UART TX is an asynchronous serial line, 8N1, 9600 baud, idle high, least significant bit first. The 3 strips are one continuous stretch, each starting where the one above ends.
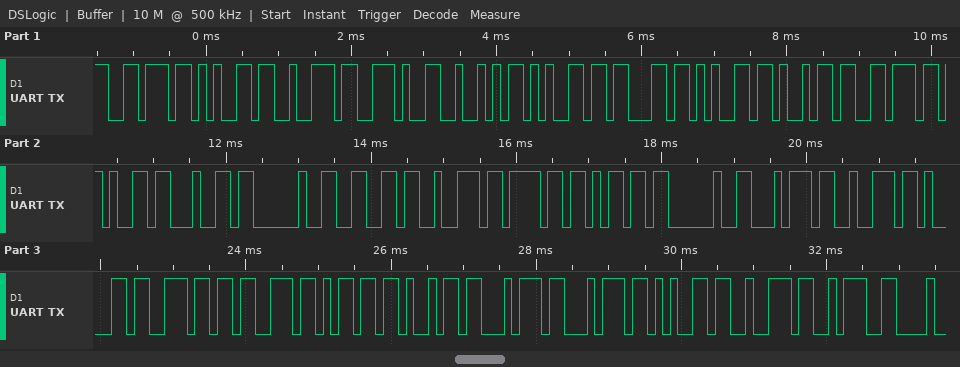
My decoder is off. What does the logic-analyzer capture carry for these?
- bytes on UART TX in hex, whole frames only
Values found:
76 65 72 2E 52 65 63 65 69 76 65 64 20 66 72 6F 6D 20 74 72 61 6E 73 6D 69 74 74 65 72 3A
